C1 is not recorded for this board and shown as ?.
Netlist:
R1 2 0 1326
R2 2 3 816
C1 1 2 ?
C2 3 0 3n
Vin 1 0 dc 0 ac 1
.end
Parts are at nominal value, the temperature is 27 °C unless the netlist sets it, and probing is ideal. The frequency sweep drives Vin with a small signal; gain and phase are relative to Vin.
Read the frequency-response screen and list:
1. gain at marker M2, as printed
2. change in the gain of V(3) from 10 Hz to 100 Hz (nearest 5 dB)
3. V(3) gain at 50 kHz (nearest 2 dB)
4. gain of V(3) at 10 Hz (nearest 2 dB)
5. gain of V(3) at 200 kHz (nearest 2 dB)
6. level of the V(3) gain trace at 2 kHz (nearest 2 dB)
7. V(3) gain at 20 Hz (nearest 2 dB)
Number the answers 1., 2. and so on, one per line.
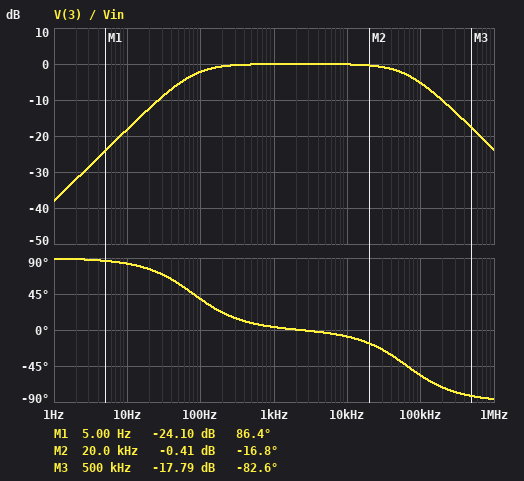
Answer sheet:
1. -0.41 dB
2. 15 dB
3. -2 dB
4. -18 dB
5. -10 dB
6. 0 dB
7. -12 dB
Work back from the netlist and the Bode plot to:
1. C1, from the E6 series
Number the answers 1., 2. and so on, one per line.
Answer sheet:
1. 1.5 µF
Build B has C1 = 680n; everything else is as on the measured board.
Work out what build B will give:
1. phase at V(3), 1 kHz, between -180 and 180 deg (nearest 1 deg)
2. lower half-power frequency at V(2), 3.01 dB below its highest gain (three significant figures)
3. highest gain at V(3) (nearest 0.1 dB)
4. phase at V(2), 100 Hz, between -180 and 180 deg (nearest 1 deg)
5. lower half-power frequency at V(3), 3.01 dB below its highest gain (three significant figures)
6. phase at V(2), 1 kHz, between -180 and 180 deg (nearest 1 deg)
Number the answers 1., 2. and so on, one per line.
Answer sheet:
1. 9 deg
2. 177 Hz
3. -0.1 dB
4. 60 deg
5. 175 Hz
6. 10 deg
